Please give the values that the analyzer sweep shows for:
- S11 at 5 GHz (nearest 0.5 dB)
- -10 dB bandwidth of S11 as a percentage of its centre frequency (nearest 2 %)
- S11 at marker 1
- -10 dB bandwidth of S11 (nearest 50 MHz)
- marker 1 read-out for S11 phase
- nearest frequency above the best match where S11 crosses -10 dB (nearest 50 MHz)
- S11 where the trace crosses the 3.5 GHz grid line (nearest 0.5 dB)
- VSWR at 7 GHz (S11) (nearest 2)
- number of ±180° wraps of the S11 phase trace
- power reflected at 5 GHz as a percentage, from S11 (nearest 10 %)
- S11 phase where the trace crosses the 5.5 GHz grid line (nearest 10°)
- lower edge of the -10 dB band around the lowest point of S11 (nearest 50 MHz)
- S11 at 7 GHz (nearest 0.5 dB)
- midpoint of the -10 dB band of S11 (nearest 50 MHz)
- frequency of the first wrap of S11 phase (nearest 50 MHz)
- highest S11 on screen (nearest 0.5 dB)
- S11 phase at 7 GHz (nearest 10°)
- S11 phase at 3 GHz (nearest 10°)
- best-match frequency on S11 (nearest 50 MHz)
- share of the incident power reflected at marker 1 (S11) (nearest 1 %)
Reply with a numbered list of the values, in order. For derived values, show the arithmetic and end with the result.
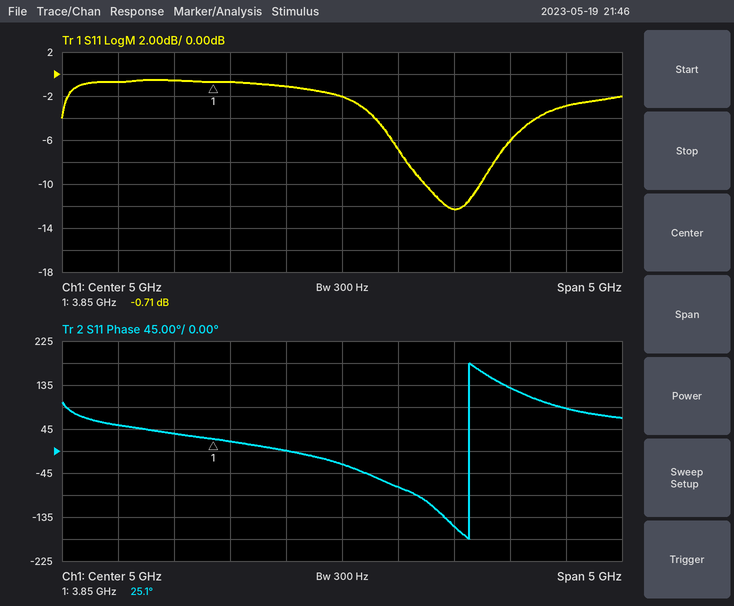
1. -2.0 dB
2. 500 MHz / 6 GHz ≈ 8 %
3. -0.71 dB
4. 6.25 GHz − 5.75 GHz = 500 MHz
5. 25.1°
6. 6.25 GHz
7. -0.5 dB
8. |Γ| = 10^(-3/20) = 0.7079; VSWR = (1 + 0.7079)/(1 − 0.7079) ≈ 6
9. 1
10. 10^(-2/10) ≈ 63.1 %, so 60 % to the nearest 10 %
11. -70°
12. 5.75 GHz
13. -3.0 dB
14. 6.00 GHz
15. 6.15 GHz
16. -0.5 dB
17. 90°
18. 50°
19. 6.00 GHz
20. 10^(-0.71/10) ≈ 85 %
